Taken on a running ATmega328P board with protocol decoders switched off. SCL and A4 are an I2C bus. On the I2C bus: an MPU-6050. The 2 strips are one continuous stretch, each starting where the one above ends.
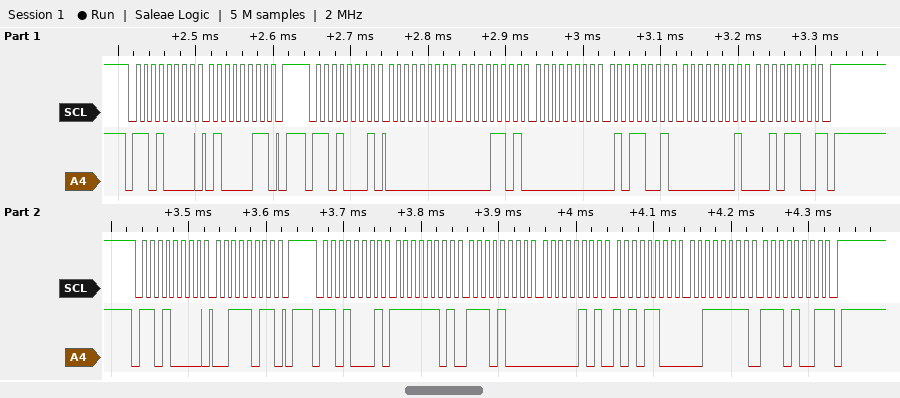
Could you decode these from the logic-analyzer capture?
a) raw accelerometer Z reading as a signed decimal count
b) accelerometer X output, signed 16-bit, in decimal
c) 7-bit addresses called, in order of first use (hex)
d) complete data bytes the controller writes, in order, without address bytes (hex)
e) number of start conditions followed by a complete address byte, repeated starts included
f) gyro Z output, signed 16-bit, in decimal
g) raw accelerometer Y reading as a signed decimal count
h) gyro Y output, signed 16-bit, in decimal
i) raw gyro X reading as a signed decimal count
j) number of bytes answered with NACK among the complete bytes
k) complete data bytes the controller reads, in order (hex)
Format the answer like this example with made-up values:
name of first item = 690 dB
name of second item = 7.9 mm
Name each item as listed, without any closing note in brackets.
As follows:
raw accelerometer Z reading as a signed decimal count = 16361
accelerometer X output, signed 16-bit, in decimal = -536
7-bit addresses called, in order of first use = 0x68
complete data bytes the controller writes, in order, without address bytes = 43 3B
number of start conditions followed by a complete address byte, repeated starts included = 4
gyro Z output, signed 16-bit, in decimal = 300
raw accelerometer Y reading as a signed decimal count = 1452
gyro Y output, signed 16-bit, in decimal = 89
raw gyro X reading as a signed decimal count = 13
number of bytes answered with NACK among the complete bytes = 2
complete data bytes the controller reads, in order = 00 0D 00 59 01 2C FD E8 05 AC 3F E9
